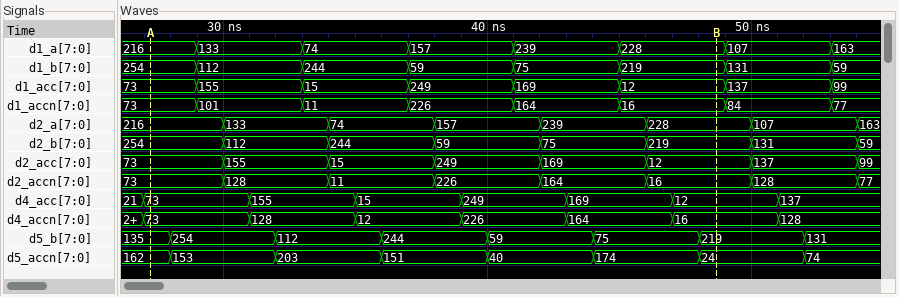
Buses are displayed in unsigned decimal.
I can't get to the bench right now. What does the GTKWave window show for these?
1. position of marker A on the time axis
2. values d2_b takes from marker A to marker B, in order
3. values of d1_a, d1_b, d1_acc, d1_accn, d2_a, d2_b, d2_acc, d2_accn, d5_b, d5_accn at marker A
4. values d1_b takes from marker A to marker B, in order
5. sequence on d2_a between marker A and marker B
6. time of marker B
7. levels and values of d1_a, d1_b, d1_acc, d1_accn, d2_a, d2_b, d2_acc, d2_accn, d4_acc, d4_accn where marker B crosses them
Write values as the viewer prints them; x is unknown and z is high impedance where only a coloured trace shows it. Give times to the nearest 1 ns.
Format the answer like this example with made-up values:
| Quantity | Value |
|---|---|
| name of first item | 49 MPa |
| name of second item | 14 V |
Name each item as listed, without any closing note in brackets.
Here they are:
| Quantity | Value |
|---|---|
| position of marker A on the time axis | 27 ns |
| values d2_b takes from marker A to marker B, in order | 254, 112, 244, 59, 75, 219 |
| values of d1_a, d1_b, d1_acc, d1_accn, d2_a, d2_b, d2_acc, d2_accn, d5_b, d5_accn at marker A | d1_a=216, d1_b=254, d1_acc=73, d1_accn=73, d2_a=216, d2_b=254, d2_acc=73, d2_accn=73, d5_b=135, d5_accn=162 |
| values d1_b takes from marker A to marker B, in order | 254, 112, 244, 59, 75, 219 |
| sequence on d2_a between marker A and marker B | 216, 133, 74, 157, 239, 228 |
| time of marker B | 49 ns |
| levels and values of d1_a, d1_b, d1_acc, d1_accn, d2_a, d2_b, d2_acc, d2_accn, d4_acc, d4_accn where marker B crosses them | d1_a=228, d1_b=219, d1_acc=12, d1_accn=16, d2_a=228, d2_b=219, d2_acc=12, d2_accn=16, d4_acc=12, d4_accn=16 |
